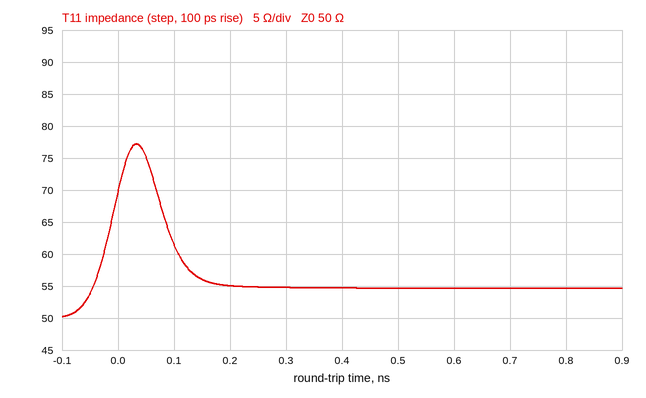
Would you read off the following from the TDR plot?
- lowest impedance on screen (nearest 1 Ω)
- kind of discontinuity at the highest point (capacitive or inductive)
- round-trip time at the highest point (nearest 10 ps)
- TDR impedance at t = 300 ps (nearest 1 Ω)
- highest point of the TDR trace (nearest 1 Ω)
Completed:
50 Ω
inductive
30 ps
55 Ω
77 Ω
